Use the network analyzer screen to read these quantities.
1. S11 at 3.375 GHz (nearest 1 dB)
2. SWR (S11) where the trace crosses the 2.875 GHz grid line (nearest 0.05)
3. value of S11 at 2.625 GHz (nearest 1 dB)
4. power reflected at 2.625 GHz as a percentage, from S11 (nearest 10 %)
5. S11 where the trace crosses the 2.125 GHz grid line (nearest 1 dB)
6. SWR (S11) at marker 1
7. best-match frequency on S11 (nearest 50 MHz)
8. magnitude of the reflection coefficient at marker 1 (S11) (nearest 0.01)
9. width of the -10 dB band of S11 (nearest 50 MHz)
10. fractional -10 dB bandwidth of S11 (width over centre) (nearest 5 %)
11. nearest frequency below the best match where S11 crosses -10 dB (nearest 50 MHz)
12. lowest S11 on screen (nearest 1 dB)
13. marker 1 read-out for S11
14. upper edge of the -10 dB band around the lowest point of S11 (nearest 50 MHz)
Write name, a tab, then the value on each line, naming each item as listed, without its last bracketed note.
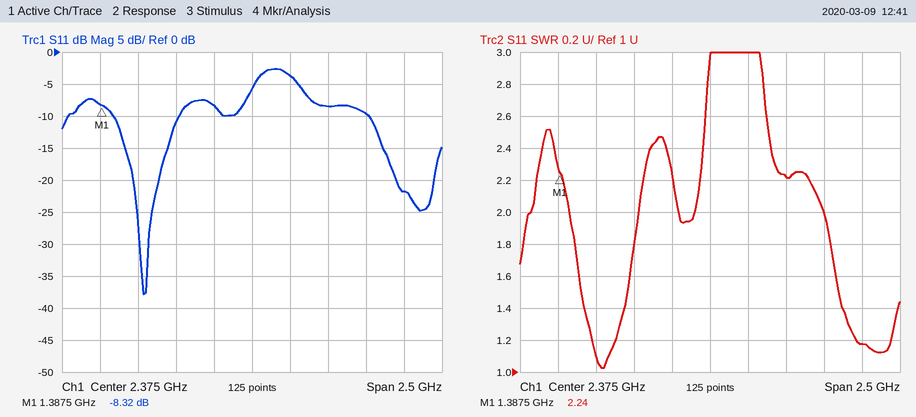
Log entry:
S11 at 3.375 GHz	-22 dB
SWR (S11) where the trace crosses the 2.875 GHz grid line	2.20
value of S11 at 2.625 GHz	-4 dB
power reflected at 2.625 GHz as a percentage, from S11	40 %
S11 where the trace crosses the 2.125 GHz grid line	-8 dB
SWR (S11) at marker 1	2.24
best-match frequency on S11	1.65 GHz
magnitude of the reflection coefficient at marker 1 (S11)	0.38
width of the -10 dB band of S11	450 MHz
fractional -10 dB bandwidth of S11 (width over centre)	25 %
nearest frequency below the best match where S11 crosses -10 dB	1.45 GHz
lowest S11 on screen	-38 dB
marker 1 read-out for S11	-8.32 dB
upper edge of the -10 dB band around the lowest point of S11	1.90 GHz
